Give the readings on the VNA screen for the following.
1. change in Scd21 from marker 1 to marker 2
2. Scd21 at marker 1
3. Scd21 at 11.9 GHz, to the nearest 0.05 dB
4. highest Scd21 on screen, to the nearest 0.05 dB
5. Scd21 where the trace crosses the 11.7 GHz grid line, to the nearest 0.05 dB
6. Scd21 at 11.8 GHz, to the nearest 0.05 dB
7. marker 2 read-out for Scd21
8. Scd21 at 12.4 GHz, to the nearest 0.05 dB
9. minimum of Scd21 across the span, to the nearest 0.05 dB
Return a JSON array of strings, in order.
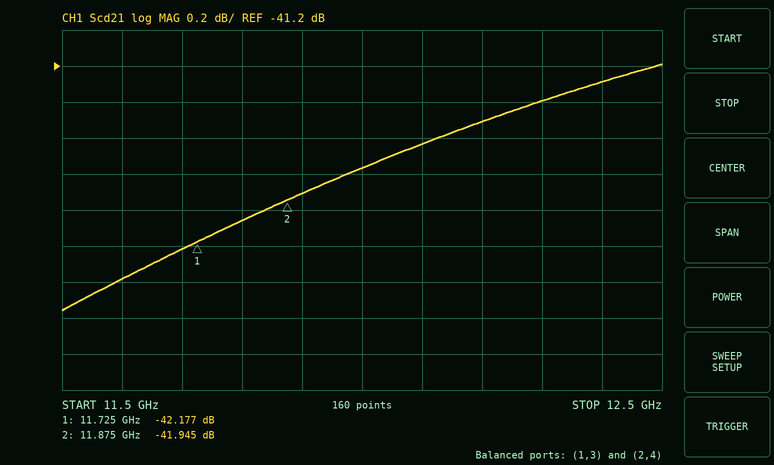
["0.232 dB", "-42.177 dB", "-41.90 dB", "-41.20 dB", "-42.20 dB", "-42.05 dB", "-41.945 dB", "-41.30 dB", "-42.55 dB"]
